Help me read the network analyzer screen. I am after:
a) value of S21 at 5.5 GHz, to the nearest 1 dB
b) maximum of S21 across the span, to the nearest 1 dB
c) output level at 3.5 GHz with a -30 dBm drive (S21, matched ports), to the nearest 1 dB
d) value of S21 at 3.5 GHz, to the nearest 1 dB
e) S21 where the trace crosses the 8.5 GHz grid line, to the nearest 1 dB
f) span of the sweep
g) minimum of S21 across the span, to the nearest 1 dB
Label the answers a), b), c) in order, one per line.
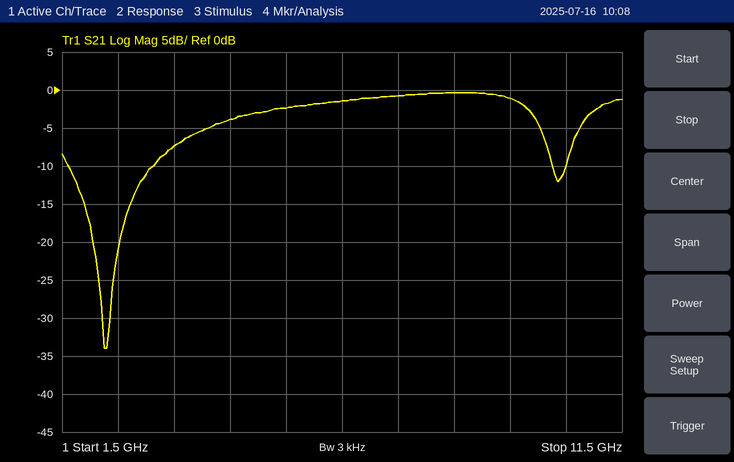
a) -2 dB
b) 0 dB
c) -37 dBm
d) -7 dB
e) 0 dB
f) 10 GHz
g) -34 dB
